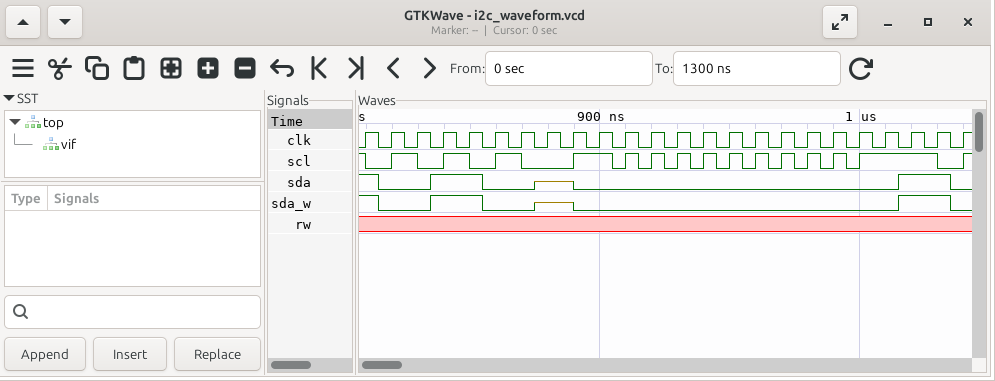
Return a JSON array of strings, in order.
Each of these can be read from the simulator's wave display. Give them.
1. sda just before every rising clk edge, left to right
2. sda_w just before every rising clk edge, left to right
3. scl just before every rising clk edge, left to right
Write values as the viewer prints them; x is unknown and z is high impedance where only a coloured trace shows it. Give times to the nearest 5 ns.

["1 0 0 1 1 0 0 z z 0 0 0 0 0 0 0 0 0 0 0 0 1 1 0", "1 0 0 1 1 0 0 z z 0 0 0 0 0 0 0 0 0 0 0 0 1 1 0", "1 0 1 0 1 0 1 0 0 1 0 0 0 0 0 0 0 0 0 0 1 1 1 0"]
